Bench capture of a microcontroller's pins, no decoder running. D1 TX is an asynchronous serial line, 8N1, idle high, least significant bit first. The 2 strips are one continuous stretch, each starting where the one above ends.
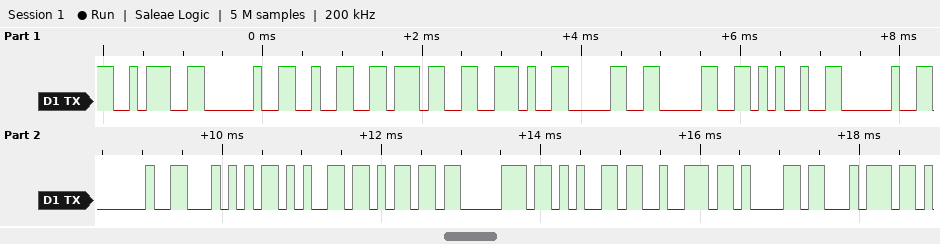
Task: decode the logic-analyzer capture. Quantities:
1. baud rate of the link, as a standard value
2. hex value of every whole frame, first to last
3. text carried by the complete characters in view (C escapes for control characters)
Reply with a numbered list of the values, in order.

1. 9600 baud
2. 0x3A 0x20 0x32 0x37 0x2E 0x30 0x30 0x25 0x20 0x20 0x54 0x65 0x6D 0x70 0x65 0x72 0x61 0x74
3. ": 27.00%  Temperat"
